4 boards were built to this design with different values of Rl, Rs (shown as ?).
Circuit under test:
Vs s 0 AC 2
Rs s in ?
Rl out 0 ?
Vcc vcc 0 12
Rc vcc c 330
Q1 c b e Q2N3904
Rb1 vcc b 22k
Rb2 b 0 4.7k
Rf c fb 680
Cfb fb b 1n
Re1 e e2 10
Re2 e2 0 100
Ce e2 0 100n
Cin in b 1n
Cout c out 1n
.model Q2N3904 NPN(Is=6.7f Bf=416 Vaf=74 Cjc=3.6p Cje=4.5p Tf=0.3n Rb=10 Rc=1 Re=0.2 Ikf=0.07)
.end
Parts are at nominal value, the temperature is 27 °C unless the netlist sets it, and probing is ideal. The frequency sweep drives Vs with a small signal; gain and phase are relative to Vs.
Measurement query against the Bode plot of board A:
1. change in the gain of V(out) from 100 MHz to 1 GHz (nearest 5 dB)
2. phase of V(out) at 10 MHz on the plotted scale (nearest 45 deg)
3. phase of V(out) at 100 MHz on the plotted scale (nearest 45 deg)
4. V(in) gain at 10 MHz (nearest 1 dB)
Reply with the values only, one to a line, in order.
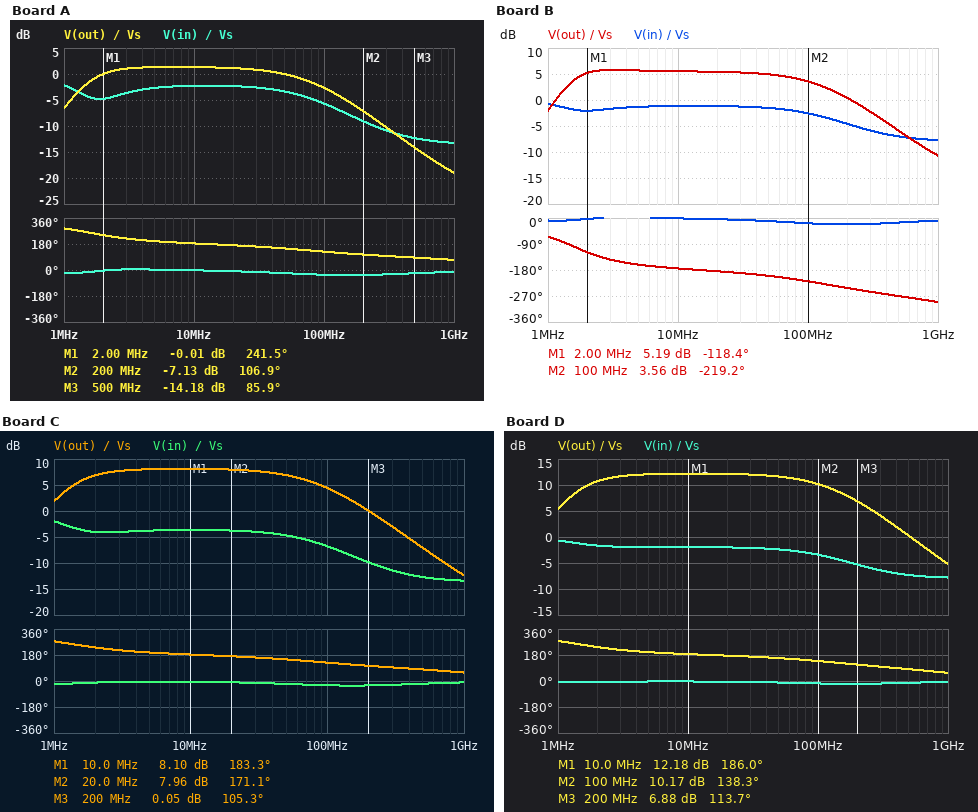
-15 dB
180 deg
135 deg
-2 dB
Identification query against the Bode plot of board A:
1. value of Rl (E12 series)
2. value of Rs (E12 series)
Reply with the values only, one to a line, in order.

22 Ω
68 Ω
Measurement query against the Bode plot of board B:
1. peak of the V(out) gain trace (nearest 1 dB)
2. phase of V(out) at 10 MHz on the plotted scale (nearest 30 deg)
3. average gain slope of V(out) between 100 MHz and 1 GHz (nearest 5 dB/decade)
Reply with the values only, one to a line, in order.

6 dB
-180 deg
-15 dB/decade
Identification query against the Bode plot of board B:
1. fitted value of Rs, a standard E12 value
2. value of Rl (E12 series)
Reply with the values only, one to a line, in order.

27 Ω
33 Ω
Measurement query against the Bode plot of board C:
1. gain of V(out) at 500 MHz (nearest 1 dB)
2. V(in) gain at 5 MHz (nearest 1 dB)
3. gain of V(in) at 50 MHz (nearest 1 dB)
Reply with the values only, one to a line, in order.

-7 dB
-4 dB
-5 dB
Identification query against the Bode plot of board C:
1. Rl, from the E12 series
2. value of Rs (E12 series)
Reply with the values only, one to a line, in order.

68 Ω
68 Ω
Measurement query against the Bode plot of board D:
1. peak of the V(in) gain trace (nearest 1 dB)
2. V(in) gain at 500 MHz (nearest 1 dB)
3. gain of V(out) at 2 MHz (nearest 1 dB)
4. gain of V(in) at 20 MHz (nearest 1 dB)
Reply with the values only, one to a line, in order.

-1 dB
-7 dB
11 dB
-2 dB
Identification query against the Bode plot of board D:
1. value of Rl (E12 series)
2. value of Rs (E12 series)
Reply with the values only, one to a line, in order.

100 Ω
27 Ω
